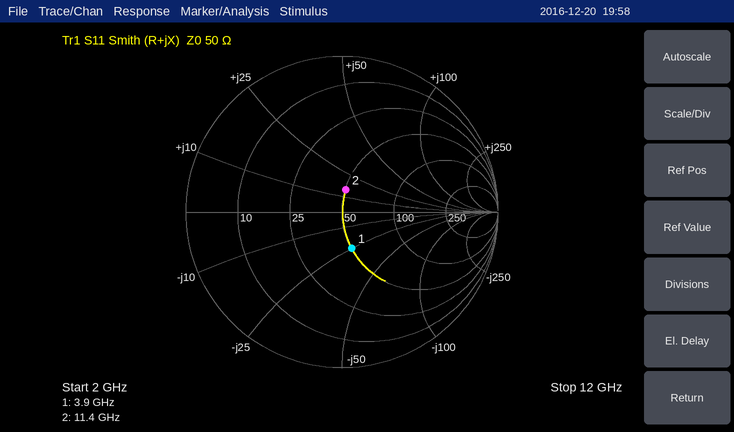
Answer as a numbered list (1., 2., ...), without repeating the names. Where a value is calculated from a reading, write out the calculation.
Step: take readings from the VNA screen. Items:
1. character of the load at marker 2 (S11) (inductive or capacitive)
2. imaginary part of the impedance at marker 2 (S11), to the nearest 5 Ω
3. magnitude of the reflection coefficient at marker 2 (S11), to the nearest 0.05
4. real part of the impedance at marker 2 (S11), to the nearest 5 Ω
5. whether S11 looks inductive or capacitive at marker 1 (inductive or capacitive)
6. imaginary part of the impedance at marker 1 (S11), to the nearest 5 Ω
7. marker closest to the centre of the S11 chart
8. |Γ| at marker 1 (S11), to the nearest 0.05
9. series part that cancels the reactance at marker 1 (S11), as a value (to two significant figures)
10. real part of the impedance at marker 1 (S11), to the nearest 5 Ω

1. inductive
2. +15 Ω
3. 0.15
4. 50 Ω
5. capacitive
6. -25 Ω
7. marker 2
8. 0.25
9. L = 25 Ω/(2π × 3.9 GHz) ≈ 1.0 nH
10. 50 Ω
